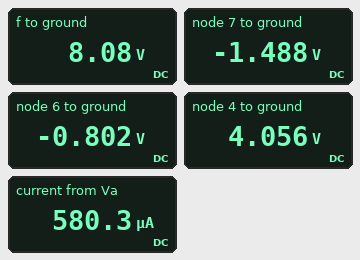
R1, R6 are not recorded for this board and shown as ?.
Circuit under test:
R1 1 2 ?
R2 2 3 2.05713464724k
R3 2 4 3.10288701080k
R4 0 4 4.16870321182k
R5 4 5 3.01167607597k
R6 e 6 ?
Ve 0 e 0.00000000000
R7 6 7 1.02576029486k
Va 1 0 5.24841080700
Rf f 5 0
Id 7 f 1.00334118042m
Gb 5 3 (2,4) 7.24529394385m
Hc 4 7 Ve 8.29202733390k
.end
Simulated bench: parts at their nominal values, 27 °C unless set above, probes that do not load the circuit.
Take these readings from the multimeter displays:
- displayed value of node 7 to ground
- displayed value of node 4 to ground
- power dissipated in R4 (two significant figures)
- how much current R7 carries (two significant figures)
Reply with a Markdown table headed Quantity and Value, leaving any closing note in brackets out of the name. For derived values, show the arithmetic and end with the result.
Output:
| Quantity | Value |
|---|---|
| displayed value of node 7 to ground | -1.488 V |
| displayed value of node 4 to ground | 4.056 V |
| power dissipated in R4 | (4.056 V)^2 / 4.169 kΩ = 3.9 mW |
| how much current R7 carries | (-802 mV - (-1.488 V)) / 1.026 kΩ = 670 µA |
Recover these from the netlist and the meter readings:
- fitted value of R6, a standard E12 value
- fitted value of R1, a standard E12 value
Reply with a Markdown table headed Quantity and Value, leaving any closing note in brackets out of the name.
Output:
| Quantity | Value |
|---|---|
| fitted value of R6, a standard E12 value | 1.2 kΩ |
| fitted value of R1, a standard E12 value | 2.2 kΩ |
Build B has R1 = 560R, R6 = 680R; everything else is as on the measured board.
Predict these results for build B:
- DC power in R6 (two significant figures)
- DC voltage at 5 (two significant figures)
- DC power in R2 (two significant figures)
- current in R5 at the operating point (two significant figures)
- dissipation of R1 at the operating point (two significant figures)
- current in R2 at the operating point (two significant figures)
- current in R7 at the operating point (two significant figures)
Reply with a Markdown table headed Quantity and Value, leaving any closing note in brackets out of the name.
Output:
| Quantity | Value |
|---|---|
| DC power in R6 | 380 µW |
| DC voltage at 5 | 9.4 V |
| DC power in R2 | 1.3 mW |
| current in R5 at the operating point | 1.5 mA |
| dissipation of R1 at the operating point | 320 µW |
| current in R2 at the operating point | 790 µA |
| current in R7 at the operating point | 750 µA |
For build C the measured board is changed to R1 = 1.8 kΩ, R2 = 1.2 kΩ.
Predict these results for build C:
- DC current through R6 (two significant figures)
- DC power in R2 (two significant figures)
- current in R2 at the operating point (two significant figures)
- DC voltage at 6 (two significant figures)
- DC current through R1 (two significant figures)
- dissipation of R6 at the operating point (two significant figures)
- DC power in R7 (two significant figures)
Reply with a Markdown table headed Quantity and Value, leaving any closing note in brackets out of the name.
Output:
| Quantity | Value |
|---|---|
| DC current through R6 | 700 µA |
| DC power in R2 | 480 µW |
| current in R2 at the operating point | 630 µA |
| DC voltage at 6 | -840 mV |
| DC current through R1 | 600 µA |
| dissipation of R6 at the operating point | 590 µW |
| DC power in R7 | 500 µW |
